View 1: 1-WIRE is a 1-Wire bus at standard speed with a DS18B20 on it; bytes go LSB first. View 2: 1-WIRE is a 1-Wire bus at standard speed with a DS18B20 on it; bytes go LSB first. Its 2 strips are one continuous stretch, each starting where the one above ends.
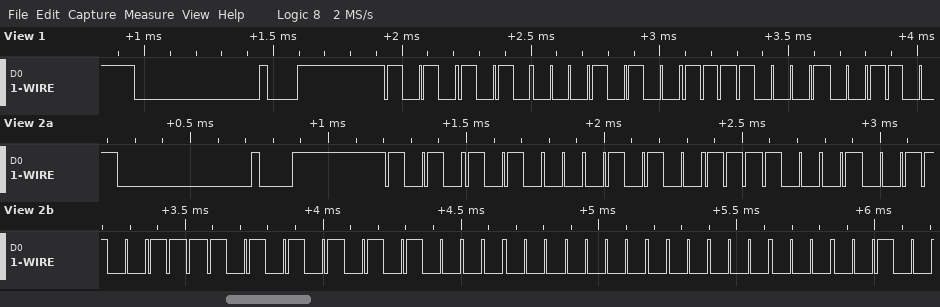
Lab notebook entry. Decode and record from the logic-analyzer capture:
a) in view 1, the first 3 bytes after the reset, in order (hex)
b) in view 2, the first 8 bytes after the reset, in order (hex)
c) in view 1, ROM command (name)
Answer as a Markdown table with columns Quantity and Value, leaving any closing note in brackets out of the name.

| Quantity | Value |
|---|---|
| in view 1, the first 3 bytes after the reset, in order | 55 28 8F |
| in view 2, the first 8 bytes after the reset, in order | 55 28 8F CC AB 0A 00 00 |
| in view 1, ROM command | Match ROM |
